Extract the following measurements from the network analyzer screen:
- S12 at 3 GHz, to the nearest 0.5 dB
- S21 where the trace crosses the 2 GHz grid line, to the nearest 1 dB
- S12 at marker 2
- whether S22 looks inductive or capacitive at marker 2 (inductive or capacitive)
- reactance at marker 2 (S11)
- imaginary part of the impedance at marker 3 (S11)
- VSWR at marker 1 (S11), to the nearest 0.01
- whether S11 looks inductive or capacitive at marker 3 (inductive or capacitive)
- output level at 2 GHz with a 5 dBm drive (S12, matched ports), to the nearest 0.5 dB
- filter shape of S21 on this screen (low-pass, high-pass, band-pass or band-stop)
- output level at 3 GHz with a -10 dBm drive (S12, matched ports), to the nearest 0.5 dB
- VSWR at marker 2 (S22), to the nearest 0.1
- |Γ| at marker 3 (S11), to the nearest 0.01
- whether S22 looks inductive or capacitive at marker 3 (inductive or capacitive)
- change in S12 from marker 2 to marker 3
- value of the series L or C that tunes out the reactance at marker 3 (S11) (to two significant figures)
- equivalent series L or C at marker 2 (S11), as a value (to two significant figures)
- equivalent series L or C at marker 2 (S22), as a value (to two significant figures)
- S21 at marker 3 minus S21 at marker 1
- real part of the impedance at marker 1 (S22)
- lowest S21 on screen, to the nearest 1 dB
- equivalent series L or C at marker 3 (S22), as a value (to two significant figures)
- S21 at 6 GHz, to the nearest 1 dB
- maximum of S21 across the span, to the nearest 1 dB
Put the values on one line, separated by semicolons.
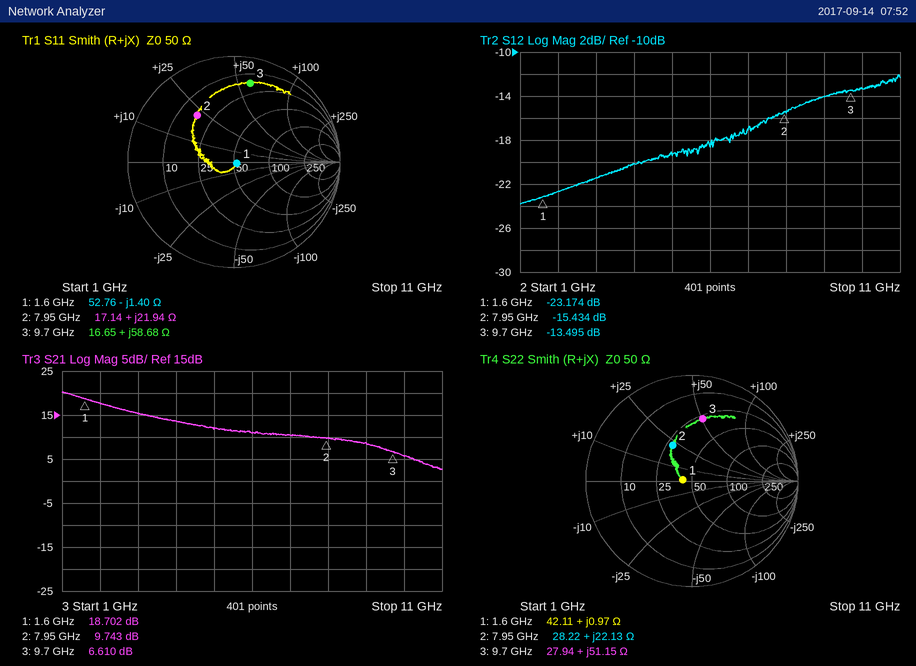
-21.5 dB; 18 dB; -15.434 dB; inductive; +21.94 Ω; +58.68 Ω; 1.06; inductive; -17.5 dBm; low-pass; -31.5 dBm; 2.2; 0.76; inductive; 1.939 dB; 280 fF; 440 pH; 440 pH; -12.092 dB; 42.11 Ω; 3 dB; 840 pH; 11 dB; 20 dB
